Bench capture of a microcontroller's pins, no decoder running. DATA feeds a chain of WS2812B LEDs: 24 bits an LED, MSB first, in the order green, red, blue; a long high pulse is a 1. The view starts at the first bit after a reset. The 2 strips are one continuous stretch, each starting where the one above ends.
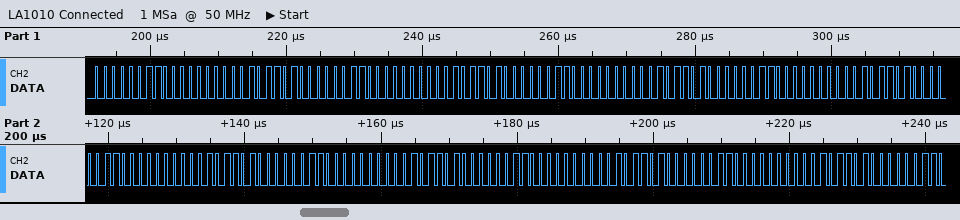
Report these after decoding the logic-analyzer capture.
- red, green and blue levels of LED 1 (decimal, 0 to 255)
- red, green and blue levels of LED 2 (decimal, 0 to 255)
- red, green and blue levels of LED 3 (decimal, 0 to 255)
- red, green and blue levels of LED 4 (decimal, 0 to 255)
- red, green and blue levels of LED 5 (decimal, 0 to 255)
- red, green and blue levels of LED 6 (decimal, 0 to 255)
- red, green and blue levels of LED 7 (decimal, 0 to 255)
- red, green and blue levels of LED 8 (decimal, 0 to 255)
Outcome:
0, 3, 45
0, 3, 45
0, 3, 45
0, 3, 45
0, 3, 45
0, 3, 45
0, 3, 45
0, 3, 45
